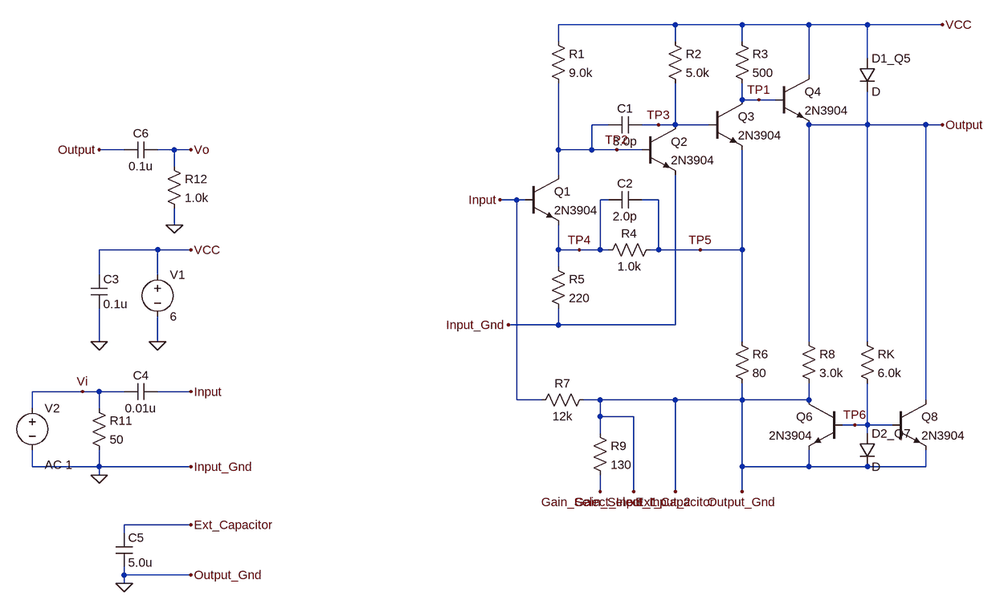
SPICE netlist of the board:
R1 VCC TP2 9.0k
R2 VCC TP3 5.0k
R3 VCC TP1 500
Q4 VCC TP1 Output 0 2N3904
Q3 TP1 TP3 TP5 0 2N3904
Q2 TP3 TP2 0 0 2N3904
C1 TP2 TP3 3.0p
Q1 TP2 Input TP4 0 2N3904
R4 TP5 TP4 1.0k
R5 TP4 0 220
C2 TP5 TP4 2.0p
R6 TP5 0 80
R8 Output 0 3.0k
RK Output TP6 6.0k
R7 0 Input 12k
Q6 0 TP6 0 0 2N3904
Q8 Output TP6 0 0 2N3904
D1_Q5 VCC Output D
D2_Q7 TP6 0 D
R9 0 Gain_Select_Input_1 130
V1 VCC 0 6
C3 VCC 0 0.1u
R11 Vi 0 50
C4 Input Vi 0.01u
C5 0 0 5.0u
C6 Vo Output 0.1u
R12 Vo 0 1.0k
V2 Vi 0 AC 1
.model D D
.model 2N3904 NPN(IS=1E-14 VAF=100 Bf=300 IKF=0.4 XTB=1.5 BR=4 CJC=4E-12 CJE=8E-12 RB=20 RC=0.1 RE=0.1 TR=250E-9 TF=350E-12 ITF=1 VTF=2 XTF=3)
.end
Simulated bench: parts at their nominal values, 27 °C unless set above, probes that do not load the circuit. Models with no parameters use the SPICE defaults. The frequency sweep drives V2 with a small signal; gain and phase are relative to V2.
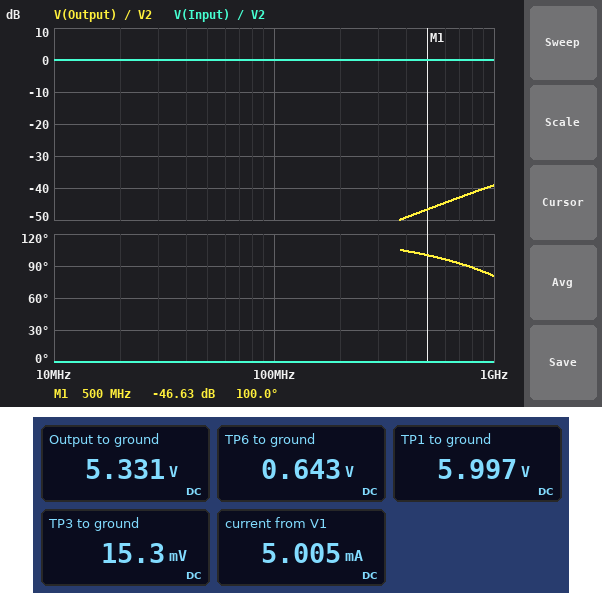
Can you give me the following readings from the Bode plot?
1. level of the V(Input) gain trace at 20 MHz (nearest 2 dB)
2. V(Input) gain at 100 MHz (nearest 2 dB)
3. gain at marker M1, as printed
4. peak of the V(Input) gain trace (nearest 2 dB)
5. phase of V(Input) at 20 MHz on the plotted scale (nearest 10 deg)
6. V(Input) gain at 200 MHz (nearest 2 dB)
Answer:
0 dB
0 dB
-46.63 dB
0 dB
0 deg
0 dB
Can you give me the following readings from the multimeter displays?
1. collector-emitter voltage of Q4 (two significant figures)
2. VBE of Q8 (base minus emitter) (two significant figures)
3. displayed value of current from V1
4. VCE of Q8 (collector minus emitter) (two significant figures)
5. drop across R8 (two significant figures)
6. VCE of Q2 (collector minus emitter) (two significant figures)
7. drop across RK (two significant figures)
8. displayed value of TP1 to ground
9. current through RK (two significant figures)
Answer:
670 mV
640 mV
5.005 mA
5.3 V
5.3 V
15 mV
4.7 V
5.997 V
780 µA
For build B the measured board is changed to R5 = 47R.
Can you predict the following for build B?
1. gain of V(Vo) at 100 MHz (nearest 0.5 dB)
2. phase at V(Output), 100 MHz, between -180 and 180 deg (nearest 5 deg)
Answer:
-68.0 dB
95 deg
